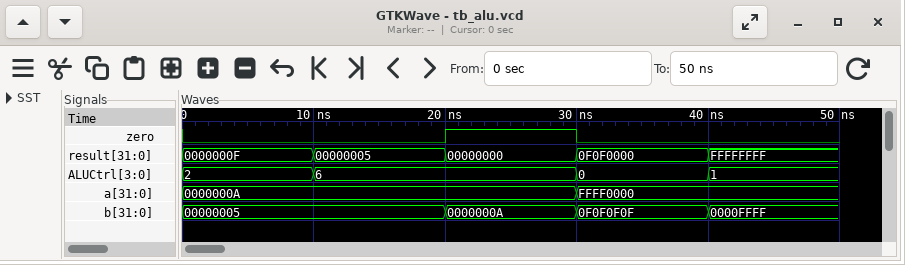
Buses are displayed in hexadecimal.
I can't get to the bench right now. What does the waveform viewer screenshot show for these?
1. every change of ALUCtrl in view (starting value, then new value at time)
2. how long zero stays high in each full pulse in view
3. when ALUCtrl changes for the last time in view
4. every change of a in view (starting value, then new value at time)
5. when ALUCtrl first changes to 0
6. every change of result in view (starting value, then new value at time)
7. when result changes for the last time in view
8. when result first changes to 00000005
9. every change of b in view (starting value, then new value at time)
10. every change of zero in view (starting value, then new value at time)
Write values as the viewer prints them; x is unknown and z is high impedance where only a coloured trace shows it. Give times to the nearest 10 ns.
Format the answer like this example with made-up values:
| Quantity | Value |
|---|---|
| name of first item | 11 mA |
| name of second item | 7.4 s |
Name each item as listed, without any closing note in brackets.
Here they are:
| Quantity | Value |
|---|---|
| every change of ALUCtrl in view | 2, 6 at 10 ns, 0 at 30 ns, 1 at 40 ns |
| how long zero stays high in each full pulse in view | 10 ns |
| when ALUCtrl changes for the last time in view | 40 ns |
| every change of a in view | 0000000A, FFFF0000 at 30 ns |
| when ALUCtrl first changes to 0 | 30 ns |
| every change of result in view | 0000000F, 00000005 at 10 ns, 00000000 at 20 ns, 0F0F0000 at 30 ns, FFFFFFFF at 40 ns |
| when result changes for the last time in view | 40 ns |
| when result first changes to 00000005 | 10 ns |
| every change of b in view | 00000005, 0000000A at 20 ns, 0F0F0F0F at 30 ns, 0000FFFF at 40 ns |
| every change of zero in view | 0, 1 at 20 ns, 0 at 30 ns |
